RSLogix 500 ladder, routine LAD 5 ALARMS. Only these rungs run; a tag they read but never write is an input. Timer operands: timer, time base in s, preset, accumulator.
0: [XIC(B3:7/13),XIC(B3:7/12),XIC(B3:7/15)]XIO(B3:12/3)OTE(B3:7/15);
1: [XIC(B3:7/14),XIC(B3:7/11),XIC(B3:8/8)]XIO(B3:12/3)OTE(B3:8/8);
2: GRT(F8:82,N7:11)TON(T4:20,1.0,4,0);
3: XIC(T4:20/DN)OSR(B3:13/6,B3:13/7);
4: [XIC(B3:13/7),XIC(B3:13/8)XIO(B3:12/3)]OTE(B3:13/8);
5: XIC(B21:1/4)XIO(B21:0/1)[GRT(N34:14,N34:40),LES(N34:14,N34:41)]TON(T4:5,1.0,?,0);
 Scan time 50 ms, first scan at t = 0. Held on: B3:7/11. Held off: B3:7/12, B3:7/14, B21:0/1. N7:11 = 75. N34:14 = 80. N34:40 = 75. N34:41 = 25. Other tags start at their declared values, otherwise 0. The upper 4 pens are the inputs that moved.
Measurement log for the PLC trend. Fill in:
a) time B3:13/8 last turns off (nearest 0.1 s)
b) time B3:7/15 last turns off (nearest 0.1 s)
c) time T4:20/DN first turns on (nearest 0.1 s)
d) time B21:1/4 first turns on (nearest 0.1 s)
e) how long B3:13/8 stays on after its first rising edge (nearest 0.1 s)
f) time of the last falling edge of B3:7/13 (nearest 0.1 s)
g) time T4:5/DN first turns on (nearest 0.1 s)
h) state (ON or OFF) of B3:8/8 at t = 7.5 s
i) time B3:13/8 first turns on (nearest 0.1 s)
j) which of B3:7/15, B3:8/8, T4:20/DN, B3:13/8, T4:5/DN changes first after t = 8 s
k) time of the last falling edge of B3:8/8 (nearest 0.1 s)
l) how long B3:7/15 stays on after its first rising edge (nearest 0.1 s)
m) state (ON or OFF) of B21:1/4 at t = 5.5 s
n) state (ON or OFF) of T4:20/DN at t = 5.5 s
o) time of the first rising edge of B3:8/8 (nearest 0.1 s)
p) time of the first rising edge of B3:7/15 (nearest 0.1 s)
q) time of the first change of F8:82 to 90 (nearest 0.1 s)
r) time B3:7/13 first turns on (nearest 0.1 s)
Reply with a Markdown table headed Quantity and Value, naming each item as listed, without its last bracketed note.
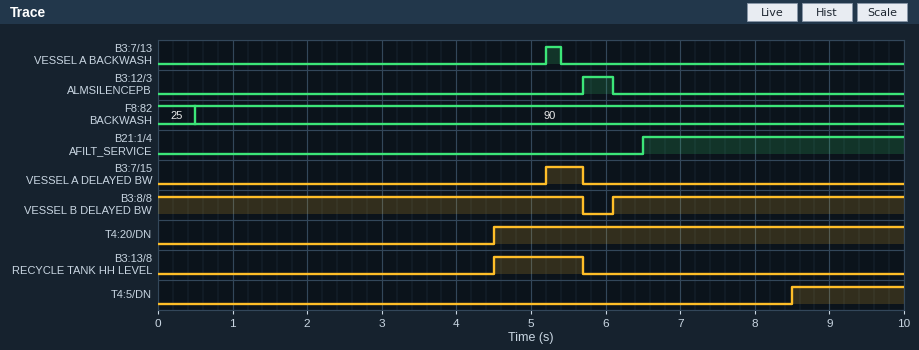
| Quantity | Value |
|---|---|
| time B3:13/8 last turns off | 5.7 s |
| time B3:7/15 last turns off | 5.7 s |
| time T4:20/DN first turns on | 4.5 s |
| time B21:1/4 first turns on | 6.5 s |
| how long B3:13/8 stays on after its first rising edge | 1.2 s |
| time of the last falling edge of B3:7/13 | 5.4 s |
| time T4:5/DN first turns on | 8.5 s |
| state (ON or OFF) of B3:8/8 at t = 7.5 s | ON |
| time B3:13/8 first turns on | 4.5 s |
| which of B3:7/15, B3:8/8, T4:20/DN, B3:13/8, T4:5/DN changes first after t = 8 s | T4:5/DN |
| time of the last falling edge of B3:8/8 | 5.7 s |
| how long B3:7/15 stays on after its first rising edge | 0.5 s |
| state (ON or OFF) of B21:1/4 at t = 5.5 s | OFF |
| state (ON or OFF) of T4:20/DN at t = 5.5 s | ON |
| time of the first rising edge of B3:8/8 | 6.1 s |
| time of the first rising edge of B3:7/15 | 5.2 s |
| time of the first change of F8:82 to 90 | 0.5 s |
| time B3:7/13 first turns on | 5.2 s |
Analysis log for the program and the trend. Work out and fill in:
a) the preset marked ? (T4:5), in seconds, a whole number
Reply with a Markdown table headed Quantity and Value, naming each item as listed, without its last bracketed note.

| Quantity | Value |
|---|---|
| the preset marked ? (T4:5), in seconds, a whole number | 2 s |
